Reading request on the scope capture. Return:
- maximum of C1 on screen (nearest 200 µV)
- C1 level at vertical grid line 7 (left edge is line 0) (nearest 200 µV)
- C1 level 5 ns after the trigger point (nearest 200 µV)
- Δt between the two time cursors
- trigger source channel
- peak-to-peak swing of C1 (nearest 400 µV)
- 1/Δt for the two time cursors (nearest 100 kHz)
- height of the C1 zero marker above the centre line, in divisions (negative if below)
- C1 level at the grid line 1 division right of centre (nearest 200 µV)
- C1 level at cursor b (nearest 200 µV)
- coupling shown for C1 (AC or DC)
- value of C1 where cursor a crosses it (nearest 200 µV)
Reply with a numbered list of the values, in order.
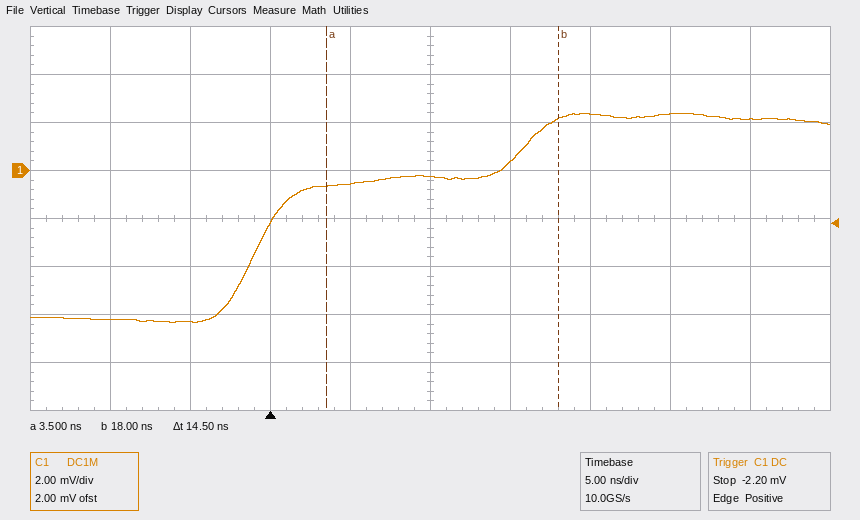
1. 2.4 mV
2. 2.4 mV
3. -600 µV
4. 14.5 ns
5. C1
6. 8.8 mV
7. 69.0 MHz
8. +1.0 div
9. 400 µV
10. 2.2 mV
11. DC
12. -600 µV
